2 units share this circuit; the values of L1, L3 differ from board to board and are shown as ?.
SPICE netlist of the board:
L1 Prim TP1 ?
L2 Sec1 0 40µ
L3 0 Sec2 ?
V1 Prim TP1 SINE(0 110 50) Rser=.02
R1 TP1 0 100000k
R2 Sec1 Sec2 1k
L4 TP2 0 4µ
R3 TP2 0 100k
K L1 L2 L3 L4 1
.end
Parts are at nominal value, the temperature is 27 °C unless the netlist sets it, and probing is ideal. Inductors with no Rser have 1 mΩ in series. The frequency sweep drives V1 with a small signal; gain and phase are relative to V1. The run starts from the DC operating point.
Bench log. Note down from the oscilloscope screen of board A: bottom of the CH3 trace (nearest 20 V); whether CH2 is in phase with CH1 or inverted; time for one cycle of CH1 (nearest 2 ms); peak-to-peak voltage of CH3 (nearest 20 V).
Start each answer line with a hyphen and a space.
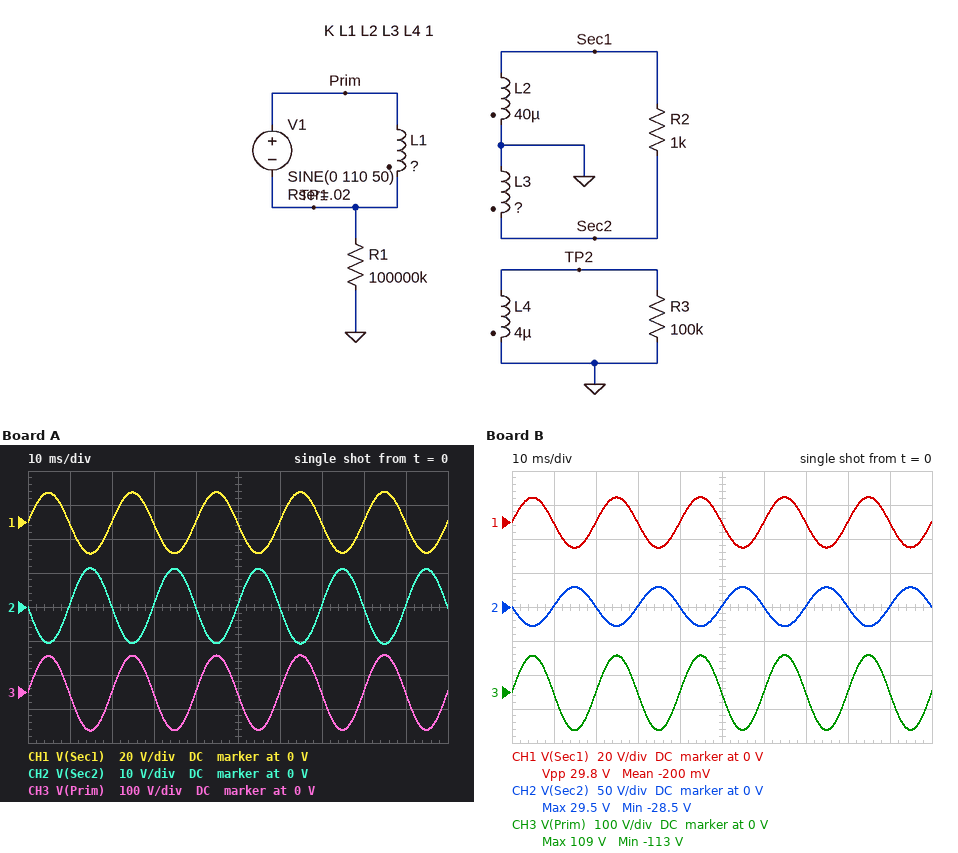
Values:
- -120 V
- inverted
- 20 ms
- 220 V
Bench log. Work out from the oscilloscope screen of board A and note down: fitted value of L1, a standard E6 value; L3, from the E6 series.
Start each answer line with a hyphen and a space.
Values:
- 1.5 mH
- 15 µH
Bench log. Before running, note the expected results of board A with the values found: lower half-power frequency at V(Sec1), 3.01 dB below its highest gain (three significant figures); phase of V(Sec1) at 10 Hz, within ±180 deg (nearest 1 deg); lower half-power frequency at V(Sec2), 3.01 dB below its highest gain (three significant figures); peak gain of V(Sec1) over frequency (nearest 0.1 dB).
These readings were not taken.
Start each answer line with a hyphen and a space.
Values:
- 2.23 Hz
- 13 deg
- 2.23 Hz
- -15.7 dB
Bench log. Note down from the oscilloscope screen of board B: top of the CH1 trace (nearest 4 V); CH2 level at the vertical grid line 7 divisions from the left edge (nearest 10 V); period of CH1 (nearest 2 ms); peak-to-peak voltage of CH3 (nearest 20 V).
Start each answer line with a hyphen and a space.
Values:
- 16 V
- 0 V
- 20 ms
- 220 V
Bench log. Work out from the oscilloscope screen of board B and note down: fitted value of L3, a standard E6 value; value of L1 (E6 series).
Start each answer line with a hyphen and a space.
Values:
- 150 µH
- 2.2 mH
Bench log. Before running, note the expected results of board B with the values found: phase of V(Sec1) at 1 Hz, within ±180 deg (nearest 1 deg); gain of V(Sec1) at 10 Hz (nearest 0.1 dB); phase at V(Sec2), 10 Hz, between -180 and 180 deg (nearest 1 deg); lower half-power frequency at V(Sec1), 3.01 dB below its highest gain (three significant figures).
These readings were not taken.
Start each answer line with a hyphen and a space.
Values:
- 57 deg
- -17.5 dB
- -171 deg
- 1.52 Hz
